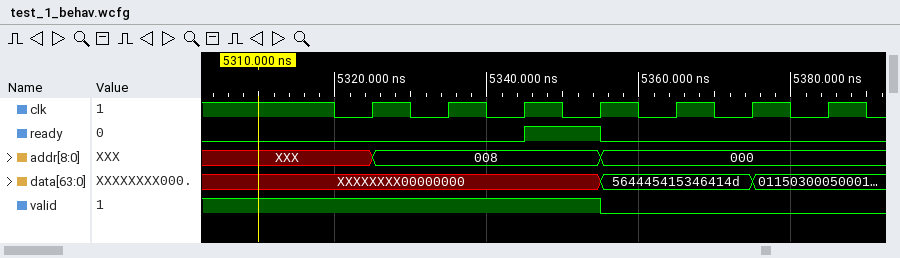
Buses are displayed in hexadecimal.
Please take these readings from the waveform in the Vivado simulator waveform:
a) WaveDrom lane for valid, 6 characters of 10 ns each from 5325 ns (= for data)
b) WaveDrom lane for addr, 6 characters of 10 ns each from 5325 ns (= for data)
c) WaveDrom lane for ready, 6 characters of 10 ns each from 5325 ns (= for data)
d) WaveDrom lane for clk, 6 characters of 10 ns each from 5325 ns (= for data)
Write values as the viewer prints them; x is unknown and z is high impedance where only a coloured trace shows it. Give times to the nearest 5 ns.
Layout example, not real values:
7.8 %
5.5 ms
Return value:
{name: 'valid', wave: '1..0..'}
{name: 'addr', wave: '=..=..', data: '008 000'}
{name: 'ready', wave: '0.10..'}
{name: 'clk', wave: 'p.....'}
